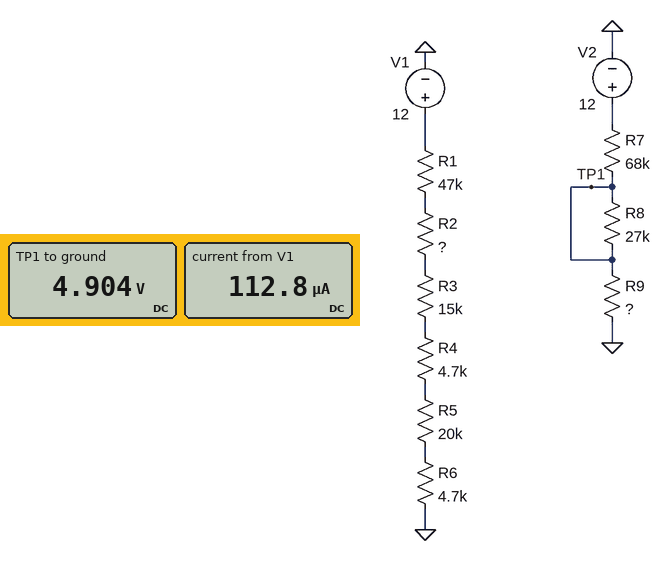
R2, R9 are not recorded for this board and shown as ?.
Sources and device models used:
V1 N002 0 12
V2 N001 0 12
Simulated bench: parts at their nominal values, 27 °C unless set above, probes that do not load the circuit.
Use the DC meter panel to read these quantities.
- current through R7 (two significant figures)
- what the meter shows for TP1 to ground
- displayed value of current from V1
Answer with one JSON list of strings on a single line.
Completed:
["100 µA", "4.904 V", "112.8 µA"]
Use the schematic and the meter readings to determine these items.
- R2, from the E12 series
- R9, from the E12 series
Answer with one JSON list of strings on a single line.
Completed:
["15 kΩ", "47 kΩ"]
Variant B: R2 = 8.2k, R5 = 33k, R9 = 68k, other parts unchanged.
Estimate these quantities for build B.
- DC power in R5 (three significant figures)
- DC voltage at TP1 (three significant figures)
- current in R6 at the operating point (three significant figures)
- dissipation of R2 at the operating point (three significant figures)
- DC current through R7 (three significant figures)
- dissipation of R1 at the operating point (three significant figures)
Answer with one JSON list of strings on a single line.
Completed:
["375 µW", "6.00 V", "107 µA", "93.1 µW", "88.2 µA", "534 µW"]
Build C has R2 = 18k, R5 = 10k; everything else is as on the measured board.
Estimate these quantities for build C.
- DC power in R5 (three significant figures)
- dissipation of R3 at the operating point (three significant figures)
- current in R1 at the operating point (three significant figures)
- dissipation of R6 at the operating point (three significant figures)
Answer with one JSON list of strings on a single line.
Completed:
["146 µW", "219 µW", "121 µA", "68.5 µW"]
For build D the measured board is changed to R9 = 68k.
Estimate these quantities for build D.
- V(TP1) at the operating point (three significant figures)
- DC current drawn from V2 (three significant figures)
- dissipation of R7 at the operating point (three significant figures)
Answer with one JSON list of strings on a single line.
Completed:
["6.00 V", "88.2 µA", "529 µW"]
